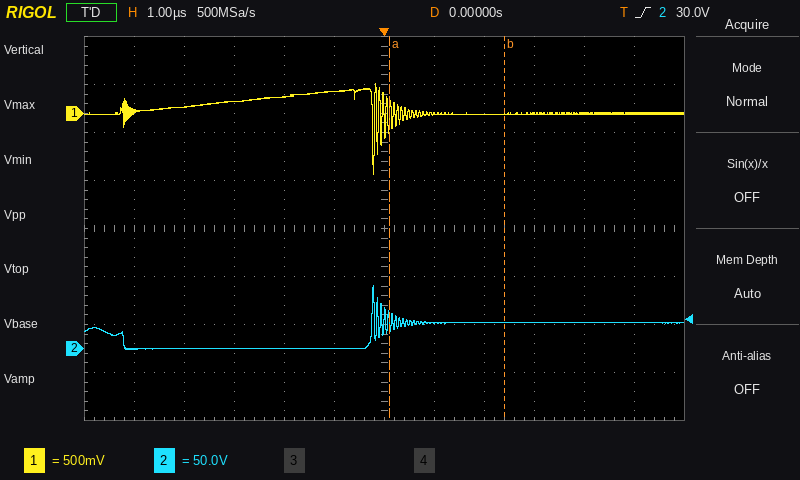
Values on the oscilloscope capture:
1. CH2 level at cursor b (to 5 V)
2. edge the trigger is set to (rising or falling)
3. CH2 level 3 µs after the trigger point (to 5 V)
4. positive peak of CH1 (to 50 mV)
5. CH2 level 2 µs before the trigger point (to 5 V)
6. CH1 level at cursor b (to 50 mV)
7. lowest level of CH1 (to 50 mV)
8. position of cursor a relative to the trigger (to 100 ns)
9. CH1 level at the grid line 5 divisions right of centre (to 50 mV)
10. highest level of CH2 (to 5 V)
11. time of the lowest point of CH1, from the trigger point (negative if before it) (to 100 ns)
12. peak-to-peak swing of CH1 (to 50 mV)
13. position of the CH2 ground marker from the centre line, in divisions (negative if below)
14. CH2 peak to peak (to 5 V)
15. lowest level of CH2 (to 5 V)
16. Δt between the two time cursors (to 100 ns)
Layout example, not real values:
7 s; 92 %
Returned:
25 V; rising; 25 V; 300 mV; 0 V; 0 mV; -650 mV; +100 ns; 0 mV; 65 V; -200 ns; 950 mV; -2.5 div; 65 V; 0 V; 2.3 µs
